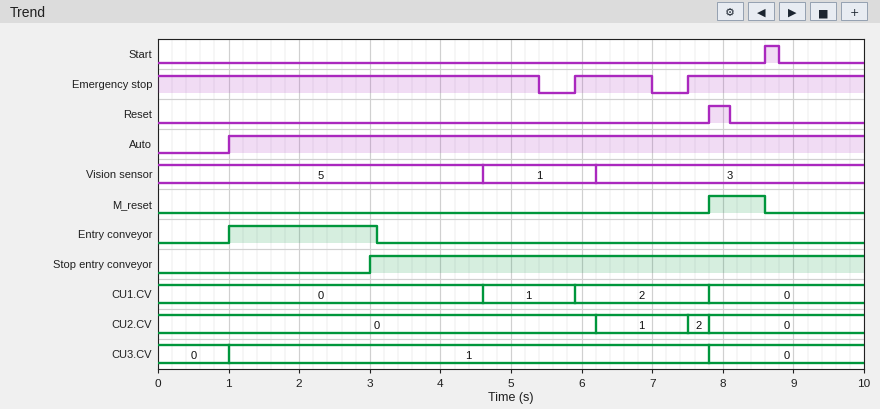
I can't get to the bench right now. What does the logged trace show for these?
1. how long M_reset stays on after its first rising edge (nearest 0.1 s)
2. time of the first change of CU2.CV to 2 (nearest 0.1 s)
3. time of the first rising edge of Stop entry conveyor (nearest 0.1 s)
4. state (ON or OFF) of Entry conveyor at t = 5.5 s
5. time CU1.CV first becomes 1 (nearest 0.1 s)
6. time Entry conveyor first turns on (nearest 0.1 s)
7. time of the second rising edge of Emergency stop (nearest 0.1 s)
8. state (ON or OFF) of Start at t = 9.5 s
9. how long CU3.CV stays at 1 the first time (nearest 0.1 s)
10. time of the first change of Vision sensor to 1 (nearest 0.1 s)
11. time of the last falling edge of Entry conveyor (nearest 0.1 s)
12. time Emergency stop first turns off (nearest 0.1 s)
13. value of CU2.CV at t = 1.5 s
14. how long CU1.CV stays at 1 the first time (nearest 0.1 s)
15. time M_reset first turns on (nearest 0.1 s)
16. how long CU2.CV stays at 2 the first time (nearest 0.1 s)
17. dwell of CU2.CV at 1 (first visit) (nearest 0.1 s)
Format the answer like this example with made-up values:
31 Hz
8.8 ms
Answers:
0.8 s
7.5 s
3.0 s
OFF
4.6 s
1.0 s
7.5 s
OFF
6.8 s
4.6 s
3.1 s
5.4 s
0
1.3 s
7.8 s
0.3 s
1.3 s
